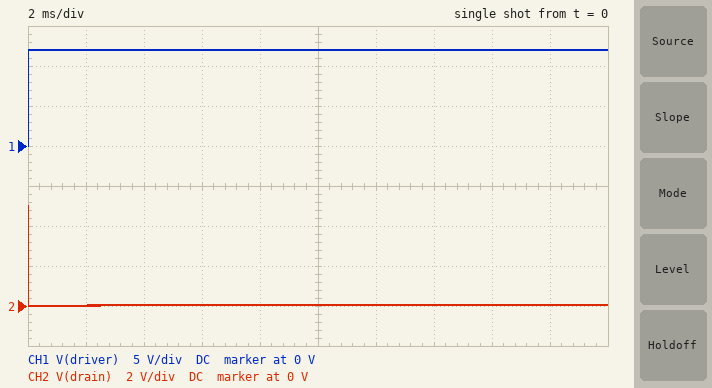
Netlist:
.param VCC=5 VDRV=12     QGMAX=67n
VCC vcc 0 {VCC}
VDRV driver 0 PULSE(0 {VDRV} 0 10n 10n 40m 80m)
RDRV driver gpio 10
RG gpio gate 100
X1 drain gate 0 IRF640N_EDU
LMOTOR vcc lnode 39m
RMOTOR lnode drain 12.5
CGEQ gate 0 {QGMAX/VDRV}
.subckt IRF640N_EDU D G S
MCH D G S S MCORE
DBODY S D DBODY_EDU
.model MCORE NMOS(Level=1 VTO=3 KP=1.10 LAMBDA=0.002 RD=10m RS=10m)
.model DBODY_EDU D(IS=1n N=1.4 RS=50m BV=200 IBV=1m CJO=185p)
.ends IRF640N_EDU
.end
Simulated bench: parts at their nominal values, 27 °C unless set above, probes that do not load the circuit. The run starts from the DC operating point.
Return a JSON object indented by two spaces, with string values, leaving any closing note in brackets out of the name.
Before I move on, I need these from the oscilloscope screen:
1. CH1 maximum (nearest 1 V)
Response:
{
  "CH1 maximum": "12 V"
}
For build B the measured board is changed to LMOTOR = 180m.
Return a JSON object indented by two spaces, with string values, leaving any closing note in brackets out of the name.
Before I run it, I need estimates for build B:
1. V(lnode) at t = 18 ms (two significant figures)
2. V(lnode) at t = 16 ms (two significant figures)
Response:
{
  "V(lnode) at t = 18 ms": "3.6 V",
  "V(lnode) at t = 16 ms": "3.4 V"
}
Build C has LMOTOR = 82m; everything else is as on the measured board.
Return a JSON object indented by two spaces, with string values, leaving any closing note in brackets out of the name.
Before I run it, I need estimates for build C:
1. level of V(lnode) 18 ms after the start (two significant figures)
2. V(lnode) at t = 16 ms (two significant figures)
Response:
{
  "level of V(lnode) 18 ms after the start": "4.7 V",
  "V(lnode) at t = 16 ms": "4.6 V"
}
